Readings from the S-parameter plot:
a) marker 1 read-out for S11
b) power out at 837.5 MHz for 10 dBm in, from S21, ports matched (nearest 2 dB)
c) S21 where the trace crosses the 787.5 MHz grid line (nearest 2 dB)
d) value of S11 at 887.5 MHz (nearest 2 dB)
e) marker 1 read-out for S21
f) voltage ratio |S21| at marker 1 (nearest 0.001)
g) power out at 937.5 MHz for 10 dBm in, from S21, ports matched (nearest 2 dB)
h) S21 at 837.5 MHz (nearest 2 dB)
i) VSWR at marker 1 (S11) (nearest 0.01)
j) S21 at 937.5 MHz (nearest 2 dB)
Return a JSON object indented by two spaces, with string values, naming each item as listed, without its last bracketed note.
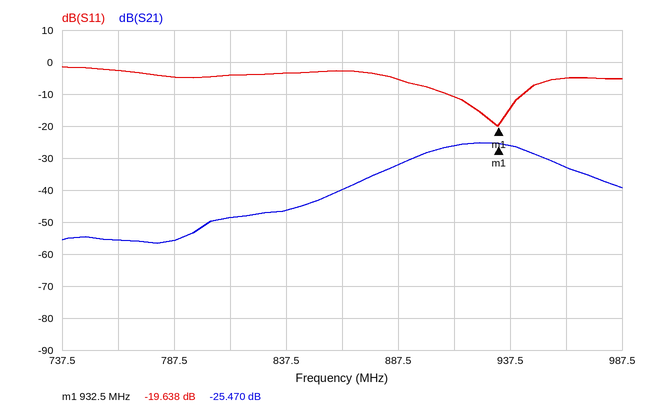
{
  "marker 1 read-out for S11": "-19.638 dB",
  "power out at 837.5 MHz for 10 dBm in, from S21, ports matched": "-36 dBm",
  "S21 where the trace crosses the 787.5 MHz grid line": "-56 dB",
  "value of S11 at 887.5 MHz": "-6 dB",
  "marker 1 read-out for S21": "-25.470 dB",
  "voltage ratio |S21| at marker 1": "0.053",
  "power out at 937.5 MHz for 10 dBm in, from S21, ports matched": "-16 dBm",
  "S21 at 837.5 MHz": "-46 dB",
  "VSWR at marker 1 (S11)": "1.23",
  "S21 at 937.5 MHz": "-26 dB"
}
